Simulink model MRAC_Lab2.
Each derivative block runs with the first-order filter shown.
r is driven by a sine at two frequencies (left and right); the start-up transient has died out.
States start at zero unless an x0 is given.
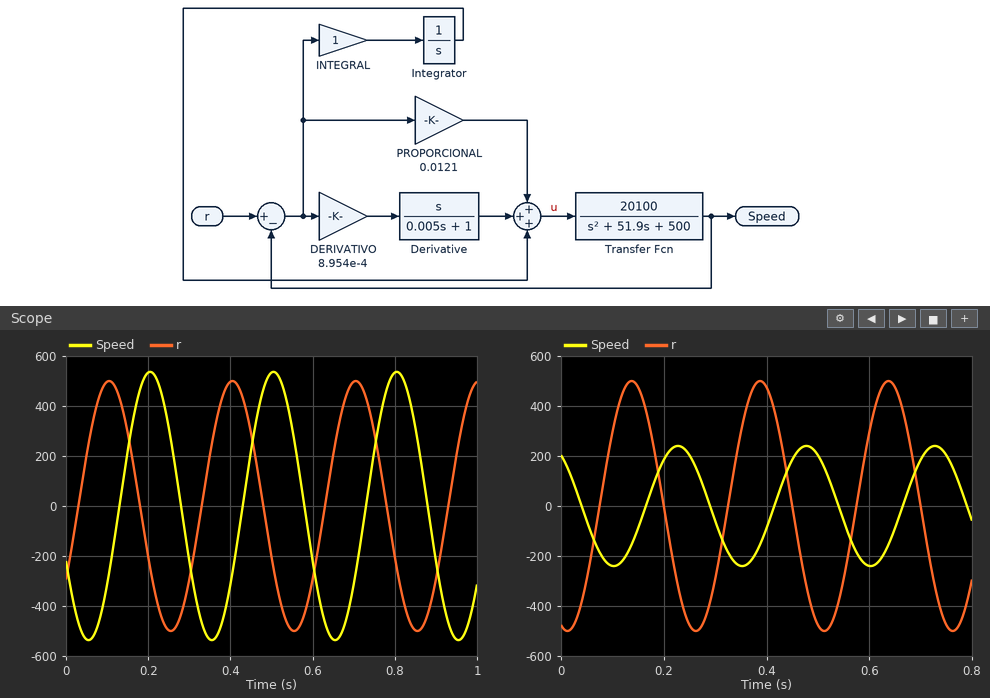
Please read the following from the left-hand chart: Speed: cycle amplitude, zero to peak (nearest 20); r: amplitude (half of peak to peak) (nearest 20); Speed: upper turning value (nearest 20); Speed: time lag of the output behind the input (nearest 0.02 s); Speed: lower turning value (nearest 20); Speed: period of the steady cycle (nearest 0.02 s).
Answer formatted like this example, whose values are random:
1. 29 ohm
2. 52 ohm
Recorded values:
1. 540
2. 500
3. 540
4. 0.10 s
5. -540
6. 0.30 s
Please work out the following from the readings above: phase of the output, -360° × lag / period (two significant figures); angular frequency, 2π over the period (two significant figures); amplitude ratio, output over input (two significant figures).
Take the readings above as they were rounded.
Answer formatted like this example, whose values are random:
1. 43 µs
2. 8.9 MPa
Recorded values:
1. -120°
2. 21 rad/s
3. 1.1
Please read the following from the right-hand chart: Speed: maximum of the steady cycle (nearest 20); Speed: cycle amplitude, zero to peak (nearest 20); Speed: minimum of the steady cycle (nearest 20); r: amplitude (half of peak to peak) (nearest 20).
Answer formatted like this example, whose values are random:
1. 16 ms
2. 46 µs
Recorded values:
1. 240
2. 240
3. -240
4. 500
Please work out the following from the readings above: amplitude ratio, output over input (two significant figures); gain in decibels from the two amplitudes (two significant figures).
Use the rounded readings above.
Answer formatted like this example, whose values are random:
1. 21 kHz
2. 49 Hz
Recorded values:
1. 0.48
2. -6.4 dB
